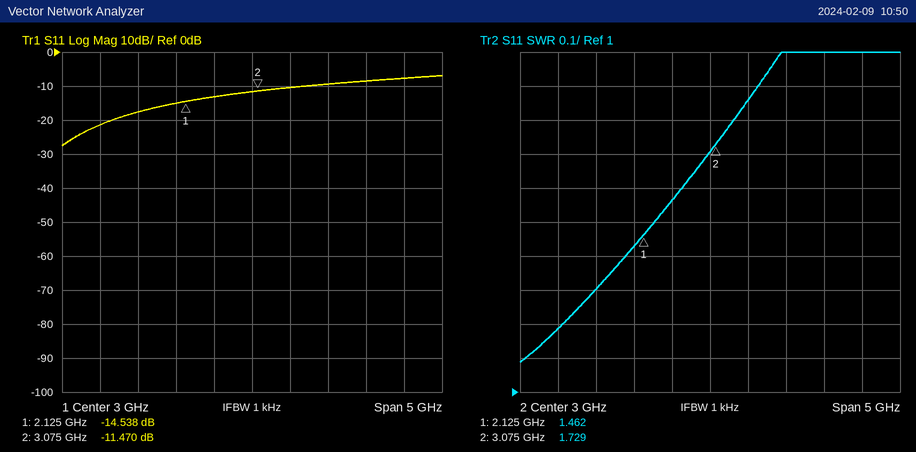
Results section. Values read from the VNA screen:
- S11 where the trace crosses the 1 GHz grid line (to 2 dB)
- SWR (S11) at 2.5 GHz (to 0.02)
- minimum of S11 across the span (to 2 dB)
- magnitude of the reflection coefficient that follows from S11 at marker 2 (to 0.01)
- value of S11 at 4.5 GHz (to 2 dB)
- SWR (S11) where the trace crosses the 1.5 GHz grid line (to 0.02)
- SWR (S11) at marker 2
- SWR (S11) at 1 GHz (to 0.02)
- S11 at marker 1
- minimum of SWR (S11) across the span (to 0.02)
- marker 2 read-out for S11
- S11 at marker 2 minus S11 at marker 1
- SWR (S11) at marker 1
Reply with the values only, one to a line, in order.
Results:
-22 dB
1.56
-28 dB
0.27
-8 dB
1.30
1.729
1.18
-14.538 dB
1.08
-11.470 dB
3.068 dB
1.462
